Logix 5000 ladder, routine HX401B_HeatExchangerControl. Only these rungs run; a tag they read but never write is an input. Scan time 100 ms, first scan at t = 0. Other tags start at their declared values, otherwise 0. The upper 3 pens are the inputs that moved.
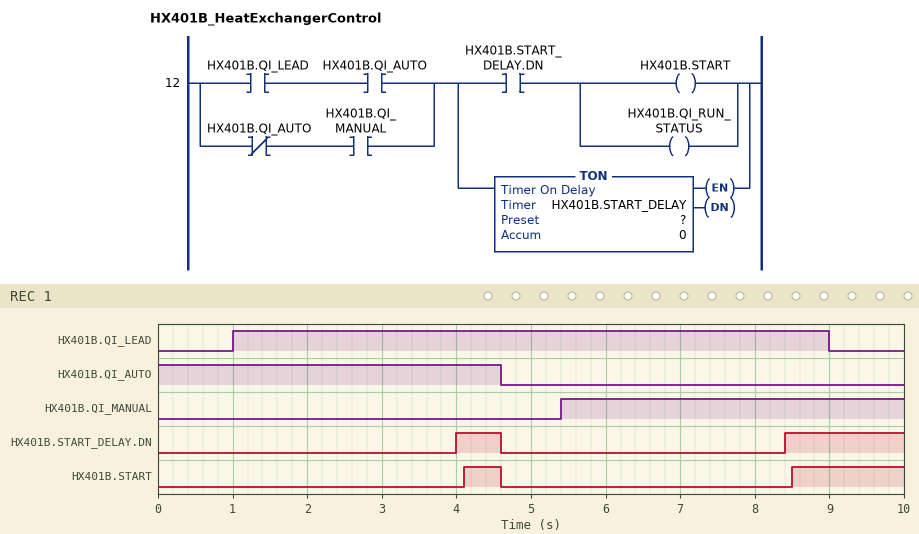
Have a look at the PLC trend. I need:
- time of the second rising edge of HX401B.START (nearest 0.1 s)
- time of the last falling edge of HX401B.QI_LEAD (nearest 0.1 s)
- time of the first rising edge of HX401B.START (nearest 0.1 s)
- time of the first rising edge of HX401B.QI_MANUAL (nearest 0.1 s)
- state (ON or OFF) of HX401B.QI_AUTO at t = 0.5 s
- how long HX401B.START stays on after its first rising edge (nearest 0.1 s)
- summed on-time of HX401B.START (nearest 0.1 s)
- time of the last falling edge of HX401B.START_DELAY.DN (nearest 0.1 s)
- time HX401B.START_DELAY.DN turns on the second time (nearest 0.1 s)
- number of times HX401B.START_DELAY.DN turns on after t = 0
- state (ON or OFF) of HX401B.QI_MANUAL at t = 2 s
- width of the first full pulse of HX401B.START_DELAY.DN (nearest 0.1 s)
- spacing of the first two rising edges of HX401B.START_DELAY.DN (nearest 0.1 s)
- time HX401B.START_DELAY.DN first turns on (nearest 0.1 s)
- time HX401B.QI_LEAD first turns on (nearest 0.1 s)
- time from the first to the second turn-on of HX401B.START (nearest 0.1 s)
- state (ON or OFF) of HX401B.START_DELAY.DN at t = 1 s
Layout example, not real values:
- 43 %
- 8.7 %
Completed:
- 8.5 s
- 9.0 s
- 4.1 s
- 5.4 s
- ON
- 0.5 s
- 2.0 s
- 4.6 s
- 8.4 s
- 2
- OFF
- 0.6 s
- 4.4 s
- 4.0 s
- 1.0 s
- 4.4 s
- OFF
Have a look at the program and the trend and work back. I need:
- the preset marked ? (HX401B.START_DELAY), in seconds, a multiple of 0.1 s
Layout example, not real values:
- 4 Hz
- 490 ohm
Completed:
- 3.0 s
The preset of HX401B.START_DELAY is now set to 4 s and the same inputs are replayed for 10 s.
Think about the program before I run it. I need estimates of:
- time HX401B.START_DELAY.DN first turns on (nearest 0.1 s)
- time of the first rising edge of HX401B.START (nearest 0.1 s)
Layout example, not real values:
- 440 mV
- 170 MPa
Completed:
- 9.4 s
- 9.5 s
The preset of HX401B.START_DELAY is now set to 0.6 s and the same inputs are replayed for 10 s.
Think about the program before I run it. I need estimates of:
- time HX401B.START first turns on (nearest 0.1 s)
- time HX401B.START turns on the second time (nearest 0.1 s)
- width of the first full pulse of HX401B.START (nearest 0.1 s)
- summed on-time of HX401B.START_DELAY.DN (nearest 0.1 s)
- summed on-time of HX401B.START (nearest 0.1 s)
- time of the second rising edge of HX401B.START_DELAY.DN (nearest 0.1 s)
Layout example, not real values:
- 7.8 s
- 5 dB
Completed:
- 1.7 s
- 6.1 s
- 2.9 s
- 7.0 s
- 6.8 s
- 6.0 s
